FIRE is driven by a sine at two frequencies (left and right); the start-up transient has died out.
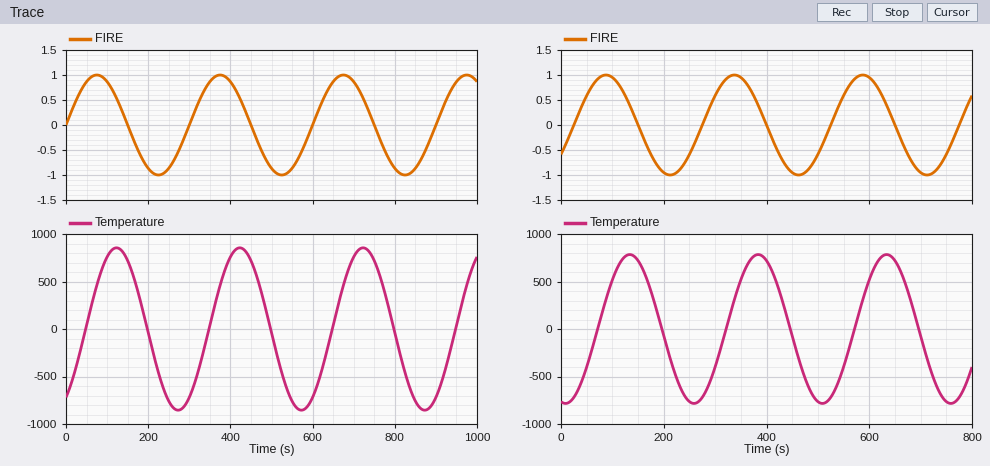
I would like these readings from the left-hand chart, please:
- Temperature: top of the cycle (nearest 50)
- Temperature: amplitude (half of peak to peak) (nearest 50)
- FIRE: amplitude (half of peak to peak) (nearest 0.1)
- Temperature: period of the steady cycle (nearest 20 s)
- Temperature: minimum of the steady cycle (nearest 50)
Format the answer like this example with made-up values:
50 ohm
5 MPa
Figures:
850
850
1.0
300 s
-850
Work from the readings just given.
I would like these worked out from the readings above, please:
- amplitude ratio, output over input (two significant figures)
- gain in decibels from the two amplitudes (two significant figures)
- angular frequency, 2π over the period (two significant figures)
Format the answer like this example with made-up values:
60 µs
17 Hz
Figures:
850
59 dB
0.021 rad/s
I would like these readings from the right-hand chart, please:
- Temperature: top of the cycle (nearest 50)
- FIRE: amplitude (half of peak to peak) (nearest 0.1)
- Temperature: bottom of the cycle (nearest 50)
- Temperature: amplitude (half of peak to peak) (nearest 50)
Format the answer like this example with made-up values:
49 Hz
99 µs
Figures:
800
1.0
-800
800
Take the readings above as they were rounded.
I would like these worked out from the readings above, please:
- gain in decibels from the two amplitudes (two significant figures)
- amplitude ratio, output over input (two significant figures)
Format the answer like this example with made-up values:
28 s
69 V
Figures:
58 dB
800
